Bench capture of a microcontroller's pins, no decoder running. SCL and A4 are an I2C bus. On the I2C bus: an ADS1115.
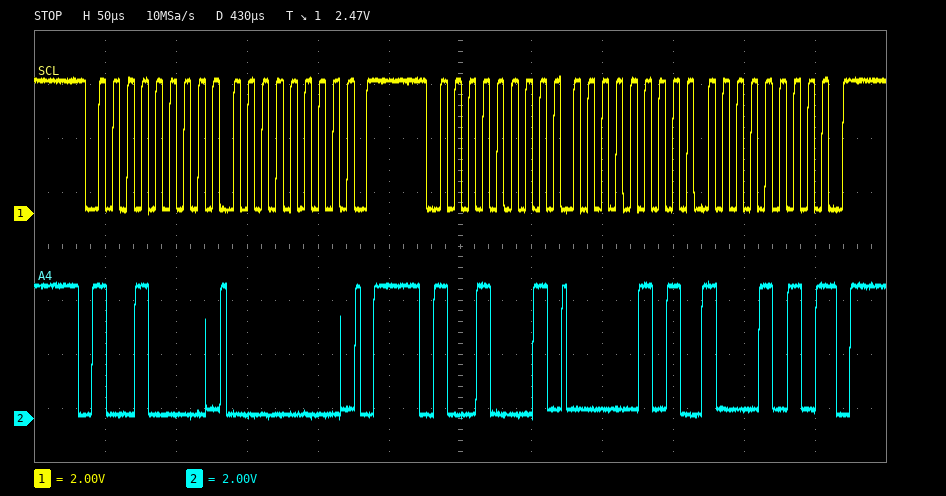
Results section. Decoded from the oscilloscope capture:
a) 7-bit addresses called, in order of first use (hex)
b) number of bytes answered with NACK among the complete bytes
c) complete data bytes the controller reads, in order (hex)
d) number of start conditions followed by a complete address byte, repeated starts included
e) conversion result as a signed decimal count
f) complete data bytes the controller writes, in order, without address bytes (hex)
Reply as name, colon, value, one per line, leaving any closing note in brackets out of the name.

7-bit addresses called, in order of first use: 0x48
number of bytes answered with NACK among the complete bytes: 1
complete data bytes the controller reads, in order: 05 8A
number of start conditions followed by a complete address byte, repeated starts included: 2
conversion result as a signed decimal count: 1418
complete data bytes the controller writes, in order, without address bytes: 00
